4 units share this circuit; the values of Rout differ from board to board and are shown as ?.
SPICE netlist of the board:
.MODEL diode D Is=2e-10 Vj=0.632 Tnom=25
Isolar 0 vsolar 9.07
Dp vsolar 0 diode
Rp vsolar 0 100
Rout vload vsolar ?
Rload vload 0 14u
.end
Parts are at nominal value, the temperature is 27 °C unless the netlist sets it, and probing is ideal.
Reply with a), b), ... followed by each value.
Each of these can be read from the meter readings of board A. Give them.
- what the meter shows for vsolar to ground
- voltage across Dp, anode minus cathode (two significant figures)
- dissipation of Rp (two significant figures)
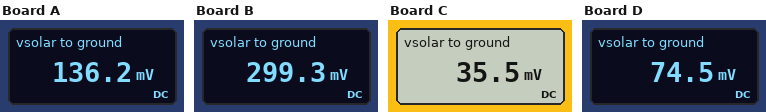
a) 136.2 mV
b) 140 mV
c) 190 µW
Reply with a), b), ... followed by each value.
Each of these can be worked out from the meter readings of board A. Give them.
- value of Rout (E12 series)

a) 0.015 Ω
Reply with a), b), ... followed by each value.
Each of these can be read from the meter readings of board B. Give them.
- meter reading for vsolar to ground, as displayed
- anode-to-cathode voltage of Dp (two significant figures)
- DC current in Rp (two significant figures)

a) 299.3 mV
b) 300 mV
c) 3.0 mA
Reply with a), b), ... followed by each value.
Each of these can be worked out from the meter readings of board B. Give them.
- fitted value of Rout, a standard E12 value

a) 0.033 Ω
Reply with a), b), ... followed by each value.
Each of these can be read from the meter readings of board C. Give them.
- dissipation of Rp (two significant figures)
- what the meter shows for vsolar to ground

a) 13 µW
b) 35.5 mV
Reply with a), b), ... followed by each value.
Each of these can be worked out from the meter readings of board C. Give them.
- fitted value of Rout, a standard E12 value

a) 3.9 mΩ
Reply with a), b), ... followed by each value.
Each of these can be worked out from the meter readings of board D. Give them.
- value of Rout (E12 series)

a) 8.2 mΩ
